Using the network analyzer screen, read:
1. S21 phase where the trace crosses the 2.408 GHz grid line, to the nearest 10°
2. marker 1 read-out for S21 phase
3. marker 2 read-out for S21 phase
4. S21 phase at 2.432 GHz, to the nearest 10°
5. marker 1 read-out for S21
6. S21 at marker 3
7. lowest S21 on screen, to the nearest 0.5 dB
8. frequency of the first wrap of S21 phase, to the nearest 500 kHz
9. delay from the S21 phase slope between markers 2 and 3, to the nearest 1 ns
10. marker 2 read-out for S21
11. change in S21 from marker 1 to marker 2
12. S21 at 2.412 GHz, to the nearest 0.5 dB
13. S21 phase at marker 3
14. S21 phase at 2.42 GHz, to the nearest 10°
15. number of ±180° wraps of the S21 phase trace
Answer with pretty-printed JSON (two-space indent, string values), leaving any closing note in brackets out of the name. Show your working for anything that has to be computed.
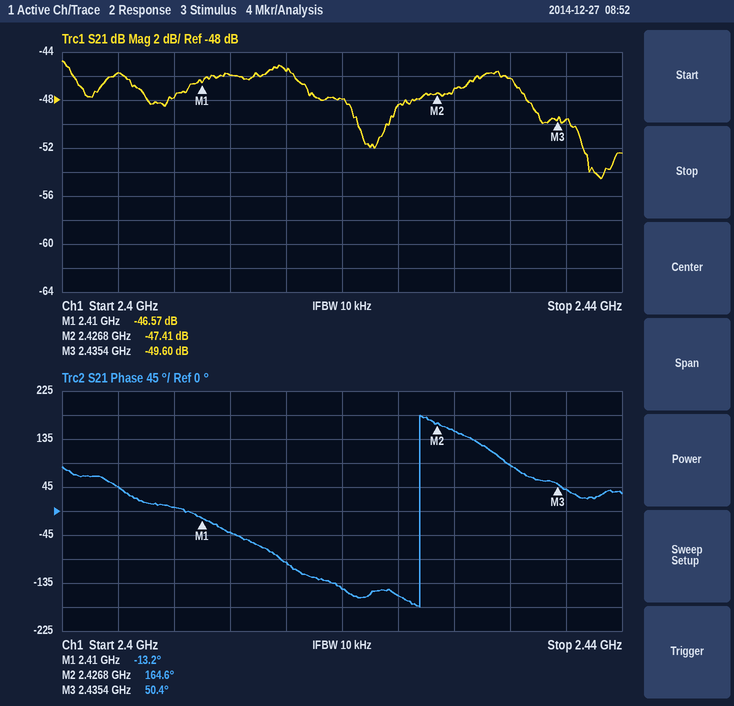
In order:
{
  "S21 phase where the trace crosses the 2.408 GHz grid line, to the nearest 10°": "10°",
  "marker 1 read-out for S21 phase": "-13.2°",
  "marker 2 read-out for S21 phase": "164.6°",
  "S21 phase at 2.432 GHz, to the nearest 10°": "90°",
  "marker 1 read-out for S21": "-46.57 dB",
  "S21 at marker 3": "-49.60 dB",
  "lowest S21 on screen, to the nearest 0.5 dB": "-54.5 dB",
  "frequency of the first wrap of S21 phase, to the nearest 500 kHz": "2.4255 GHz",
  "delay from the S21 phase slope between markers 2 and 3, to the nearest 1 ns": "−(50.4° − (164.6°))/(360° × 8.6 MHz) ≈ 37 ns",
  "marker 2 read-out for S21": "-47.41 dB",
  "change in S21 from marker 1 to marker 2": "-47.41 − (-46.57) = -0.84 dB",
  "S21 at 2.412 GHz, to the nearest 0.5 dB": "-46.0 dB",
  "S21 phase at marker 3": "50.4°",
  "S21 phase at 2.42 GHz, to the nearest 10°": "-150°",
  "number of ±180° wraps of the S21 phase trace": "1"
}
